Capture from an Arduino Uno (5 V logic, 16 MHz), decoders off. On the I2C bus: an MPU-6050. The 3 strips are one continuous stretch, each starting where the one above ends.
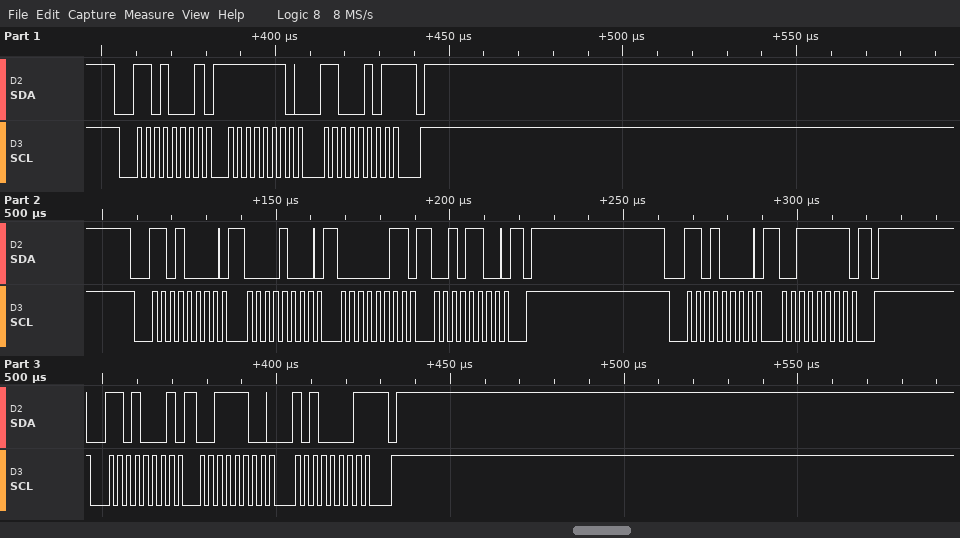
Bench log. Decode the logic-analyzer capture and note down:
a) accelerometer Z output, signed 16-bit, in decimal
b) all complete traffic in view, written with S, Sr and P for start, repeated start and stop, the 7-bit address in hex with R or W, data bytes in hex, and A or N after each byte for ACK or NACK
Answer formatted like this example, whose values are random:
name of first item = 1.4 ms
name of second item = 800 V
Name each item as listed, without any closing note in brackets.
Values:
accelerometer Z output, signed 16-bit, in decimal = 15521
all complete traffic in view, written with S, Sr and P for start, repeated start and stop, the 7-bit address in hex with R or W, data bytes in hex, and A or N after each byte for ACK or NACK = S 68R A FE A C5 N P S 68W A 08 A 03 A 2C A P S 68W A 3F A P S 68R A 3C A A1 N P
